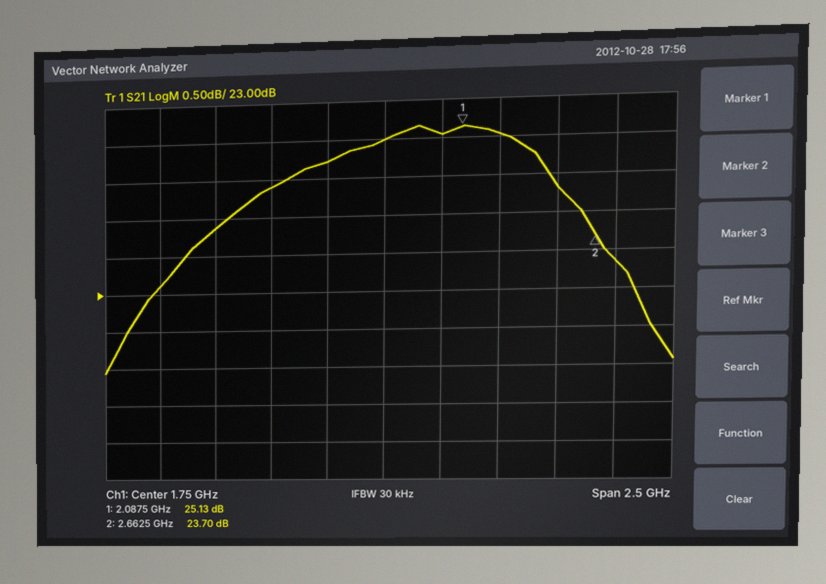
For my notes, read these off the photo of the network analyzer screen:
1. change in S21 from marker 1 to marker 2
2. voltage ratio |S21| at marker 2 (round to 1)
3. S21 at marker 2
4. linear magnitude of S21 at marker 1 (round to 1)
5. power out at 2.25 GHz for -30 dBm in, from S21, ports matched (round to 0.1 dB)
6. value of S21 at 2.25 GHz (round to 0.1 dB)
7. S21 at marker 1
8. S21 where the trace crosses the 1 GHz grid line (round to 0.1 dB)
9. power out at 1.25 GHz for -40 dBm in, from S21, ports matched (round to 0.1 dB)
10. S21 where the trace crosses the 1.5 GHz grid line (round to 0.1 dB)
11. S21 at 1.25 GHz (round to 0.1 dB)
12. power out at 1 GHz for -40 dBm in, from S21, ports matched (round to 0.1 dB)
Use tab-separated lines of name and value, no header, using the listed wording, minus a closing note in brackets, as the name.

change in S21 from marker 1 to marker 2	-1.43 dB
voltage ratio |S21| at marker 2	15
S21 at marker 2	23.70 dB
linear magnitude of S21 at marker 1	18
power out at 2.25 GHz for -30 dBm in, from S21, ports matched	-5.0 dBm
value of S21 at 2.25 GHz	25.0 dB
S21 at marker 1	25.13 dB
S21 where the trace crosses the 1 GHz grid line	23.9 dB
power out at 1.25 GHz for -40 dBm in, from S21, ports matched	-15.6 dBm
S21 where the trace crosses the 1.5 GHz grid line	24.7 dB
S21 at 1.25 GHz	24.4 dB
power out at 1 GHz for -40 dBm in, from S21, ports matched	-16.1 dBm
